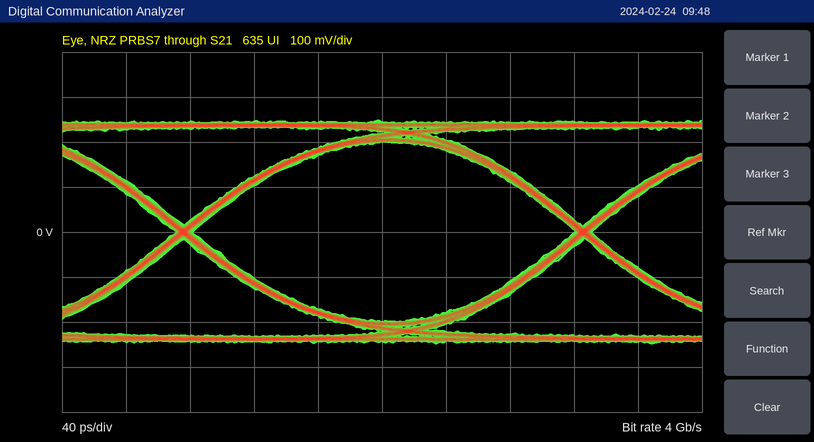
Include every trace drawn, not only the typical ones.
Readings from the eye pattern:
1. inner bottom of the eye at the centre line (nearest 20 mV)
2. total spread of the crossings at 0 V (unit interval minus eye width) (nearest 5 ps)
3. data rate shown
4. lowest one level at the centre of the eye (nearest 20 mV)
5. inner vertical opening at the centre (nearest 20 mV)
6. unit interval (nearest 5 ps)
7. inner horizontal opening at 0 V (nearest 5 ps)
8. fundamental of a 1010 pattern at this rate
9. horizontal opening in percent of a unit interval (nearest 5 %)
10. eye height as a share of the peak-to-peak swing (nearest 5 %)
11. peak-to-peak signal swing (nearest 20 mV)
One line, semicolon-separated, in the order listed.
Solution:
-200 mV; 10 ps; 4 Gb/s; 200 mV; 400 mV; 250 ps; 240 ps; 2 GHz; 95 %; 80 %; 500 mV
